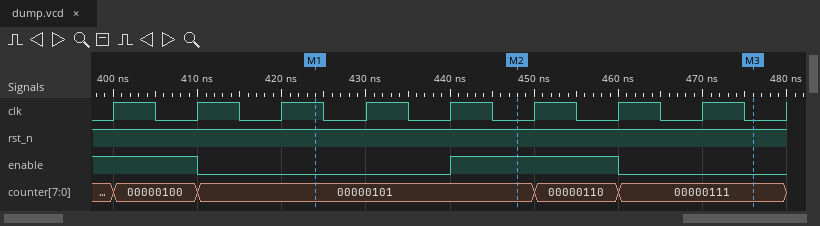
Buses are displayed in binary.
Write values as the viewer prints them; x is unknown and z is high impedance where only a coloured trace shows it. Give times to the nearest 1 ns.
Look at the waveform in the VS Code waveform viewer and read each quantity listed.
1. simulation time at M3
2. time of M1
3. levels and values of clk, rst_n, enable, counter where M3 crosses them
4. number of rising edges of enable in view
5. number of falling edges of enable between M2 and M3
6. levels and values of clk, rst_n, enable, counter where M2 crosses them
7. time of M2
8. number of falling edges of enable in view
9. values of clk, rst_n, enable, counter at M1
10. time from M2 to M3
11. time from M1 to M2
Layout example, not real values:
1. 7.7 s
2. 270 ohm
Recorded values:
1. 476 ns
2. 424 ns
3. clk=0, rst_n=1, enable=0, counter=00000111
4. 1
5. 1
6. clk=0, rst_n=1, enable=1, counter=00000101
7. 448 ns
8. 2
9. clk=1, rst_n=1, enable=0, counter=00000101
10. 28 ns
11. 24 ns
